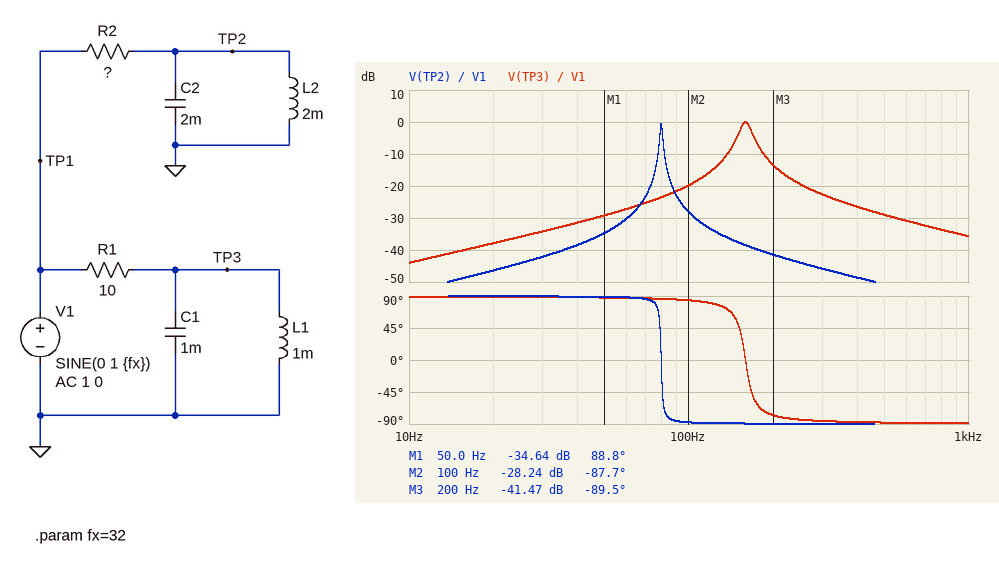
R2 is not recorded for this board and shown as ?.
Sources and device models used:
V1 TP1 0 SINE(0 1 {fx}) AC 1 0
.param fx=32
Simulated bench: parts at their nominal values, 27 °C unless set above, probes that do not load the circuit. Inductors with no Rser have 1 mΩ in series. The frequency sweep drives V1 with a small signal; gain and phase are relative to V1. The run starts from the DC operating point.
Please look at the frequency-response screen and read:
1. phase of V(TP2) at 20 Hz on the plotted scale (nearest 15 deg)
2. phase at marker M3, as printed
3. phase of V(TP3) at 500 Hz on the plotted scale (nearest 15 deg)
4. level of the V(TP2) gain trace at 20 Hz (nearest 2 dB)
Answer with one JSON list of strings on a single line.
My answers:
["90 deg", "-89.5 deg", "-90 deg", "-46 dB"]
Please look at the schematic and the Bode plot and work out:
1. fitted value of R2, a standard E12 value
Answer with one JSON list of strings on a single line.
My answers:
["56 Ω"]
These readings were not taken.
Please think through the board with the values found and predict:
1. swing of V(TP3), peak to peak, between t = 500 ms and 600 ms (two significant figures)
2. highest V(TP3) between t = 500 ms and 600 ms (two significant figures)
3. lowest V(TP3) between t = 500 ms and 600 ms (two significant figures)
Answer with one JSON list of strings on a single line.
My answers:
["42 mV", "21 mV", "-21 mV"]
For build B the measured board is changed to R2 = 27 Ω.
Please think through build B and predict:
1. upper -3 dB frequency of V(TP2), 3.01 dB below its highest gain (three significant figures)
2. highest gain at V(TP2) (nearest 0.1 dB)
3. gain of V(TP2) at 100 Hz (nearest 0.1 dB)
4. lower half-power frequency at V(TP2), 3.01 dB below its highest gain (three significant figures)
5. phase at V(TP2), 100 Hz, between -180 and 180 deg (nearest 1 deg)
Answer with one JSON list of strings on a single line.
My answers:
["81.1 Hz", "-0.2 dB", "-21.9 dB", "78.1 Hz", "-85 deg"]
